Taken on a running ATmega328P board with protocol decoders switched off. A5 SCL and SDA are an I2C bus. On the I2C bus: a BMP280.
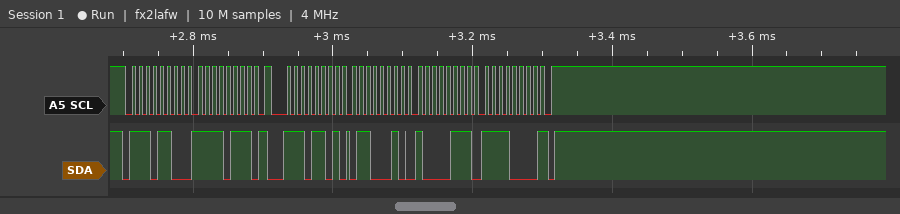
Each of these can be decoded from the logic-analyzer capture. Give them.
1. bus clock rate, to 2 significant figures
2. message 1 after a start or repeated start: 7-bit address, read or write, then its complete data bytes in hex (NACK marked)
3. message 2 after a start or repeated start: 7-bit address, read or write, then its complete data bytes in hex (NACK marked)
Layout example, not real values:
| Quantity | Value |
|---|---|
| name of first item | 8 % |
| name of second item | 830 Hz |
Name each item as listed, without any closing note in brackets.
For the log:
| Quantity | Value |
|---|---|
| bus clock rate, to 2 significant figures | 100 kHz |
| message 1 after a start or repeated start: 7-bit address, read or write, then its complete data bytes in hex | 0x76 write: F7 |
| message 2 after a start or repeated start: 7-bit address, read or write, then its complete data bytes in hex | 0x76 read: 62 87 F0 NACK |
